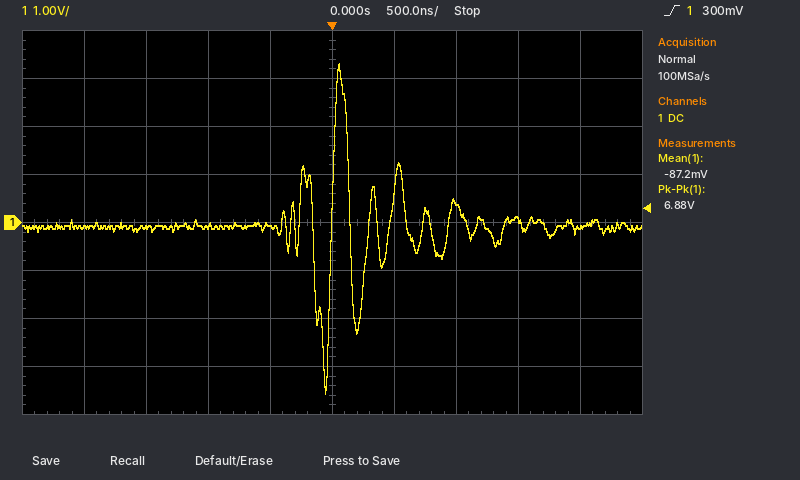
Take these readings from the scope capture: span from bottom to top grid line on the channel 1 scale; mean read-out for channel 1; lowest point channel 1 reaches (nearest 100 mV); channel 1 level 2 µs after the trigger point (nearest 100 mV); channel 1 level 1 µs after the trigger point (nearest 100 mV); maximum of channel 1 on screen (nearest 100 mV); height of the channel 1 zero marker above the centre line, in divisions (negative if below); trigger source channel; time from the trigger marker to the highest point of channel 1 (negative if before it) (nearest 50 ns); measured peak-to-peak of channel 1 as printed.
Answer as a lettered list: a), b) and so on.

a) 8 V
b) -87.2 mV
c) -3.6 V
d) -100 mV
e) 400 mV
f) 3.3 V
g) 0.0 div
h) channel 1
i) +50 ns
j) 6.88 V
